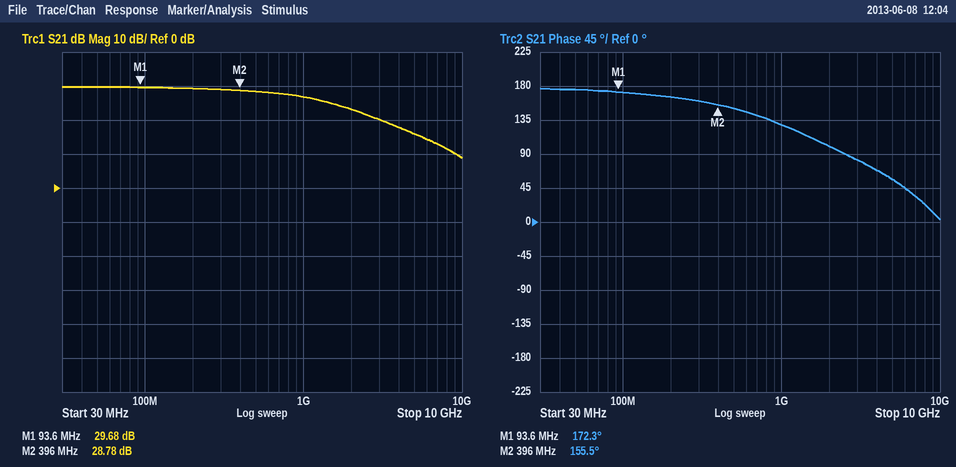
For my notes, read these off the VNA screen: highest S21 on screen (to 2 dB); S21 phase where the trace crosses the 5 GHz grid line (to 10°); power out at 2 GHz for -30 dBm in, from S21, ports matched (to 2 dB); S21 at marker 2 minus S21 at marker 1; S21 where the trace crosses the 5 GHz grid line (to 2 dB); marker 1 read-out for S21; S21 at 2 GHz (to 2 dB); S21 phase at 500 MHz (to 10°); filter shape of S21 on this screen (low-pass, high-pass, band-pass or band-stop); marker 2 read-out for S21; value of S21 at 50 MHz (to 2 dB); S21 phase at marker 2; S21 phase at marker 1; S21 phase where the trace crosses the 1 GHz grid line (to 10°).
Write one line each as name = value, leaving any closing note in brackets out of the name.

highest S21 on screen = 30 dB
S21 phase where the trace crosses the 5 GHz grid line = 60°
power out at 2 GHz for -30 dBm in, from S21, ports matched = -6 dBm
S21 at marker 2 minus S21 at marker 1 = -0.90 dB
S21 where the trace crosses the 5 GHz grid line = 16 dB
marker 1 read-out for S21 = 29.68 dB
S21 at 2 GHz = 24 dB
S21 phase at 500 MHz = 150°
filter shape of S21 on this screen = low-pass
marker 2 read-out for S21 = 28.78 dB
value of S21 at 50 MHz = 30 dB
S21 phase at marker 2 = 155.5°
S21 phase at marker 1 = 172.3°
S21 phase where the trace crosses the 1 GHz grid line = 130°
